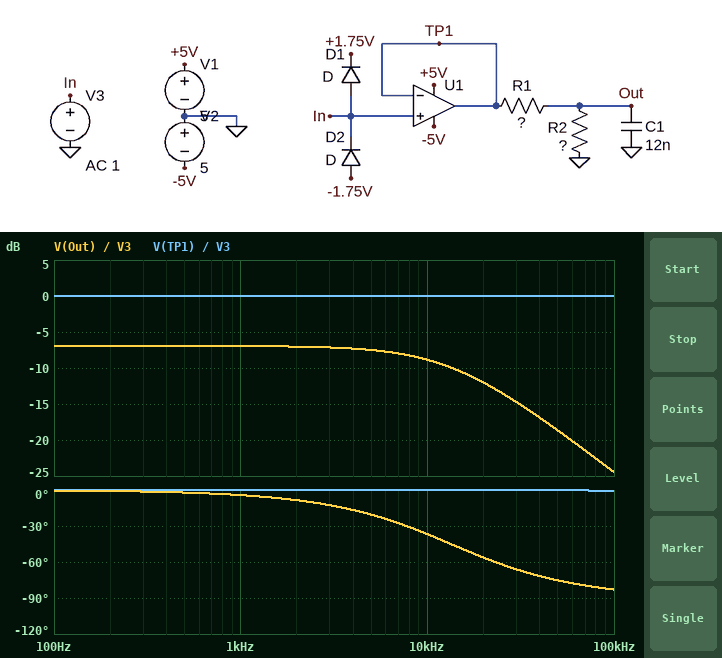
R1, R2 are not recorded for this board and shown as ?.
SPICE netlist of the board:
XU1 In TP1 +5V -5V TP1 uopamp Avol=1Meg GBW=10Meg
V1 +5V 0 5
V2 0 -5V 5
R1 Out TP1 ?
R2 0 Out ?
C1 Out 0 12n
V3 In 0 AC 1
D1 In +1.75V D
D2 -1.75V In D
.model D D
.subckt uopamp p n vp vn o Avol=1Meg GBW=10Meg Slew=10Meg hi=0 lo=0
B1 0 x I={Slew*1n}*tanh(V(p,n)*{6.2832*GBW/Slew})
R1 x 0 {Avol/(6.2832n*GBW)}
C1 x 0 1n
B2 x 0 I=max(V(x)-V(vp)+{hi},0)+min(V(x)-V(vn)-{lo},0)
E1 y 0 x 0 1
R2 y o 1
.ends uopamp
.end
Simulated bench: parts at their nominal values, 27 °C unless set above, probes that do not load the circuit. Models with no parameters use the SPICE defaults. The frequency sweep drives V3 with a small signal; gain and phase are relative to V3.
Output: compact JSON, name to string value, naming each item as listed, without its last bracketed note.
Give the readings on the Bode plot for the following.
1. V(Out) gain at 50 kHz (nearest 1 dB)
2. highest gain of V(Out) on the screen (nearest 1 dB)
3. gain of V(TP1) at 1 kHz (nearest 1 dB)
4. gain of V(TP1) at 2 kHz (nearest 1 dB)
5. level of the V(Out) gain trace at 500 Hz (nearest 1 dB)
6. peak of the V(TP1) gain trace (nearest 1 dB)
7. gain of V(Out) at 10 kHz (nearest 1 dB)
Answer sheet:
{"V(Out) gain at 50 kHz": "-19 dB", "highest gain of V(Out) on the screen": "-7 dB", "gain of V(TP1) at 1 kHz": "0 dB", "gain of V(TP1) at 2 kHz": "0 dB", "level of the V(Out) gain trace at 500 Hz": "-7 dB", "peak of the V(TP1) gain trace": "0 dB", "gain of V(Out) at 10 kHz": "-9 dB"}
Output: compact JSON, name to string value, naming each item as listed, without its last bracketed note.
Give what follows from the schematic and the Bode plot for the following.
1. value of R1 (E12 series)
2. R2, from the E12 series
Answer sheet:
{"value of R1": "2.2 kΩ", "R2, from the E12 series": "1.8 kΩ"}
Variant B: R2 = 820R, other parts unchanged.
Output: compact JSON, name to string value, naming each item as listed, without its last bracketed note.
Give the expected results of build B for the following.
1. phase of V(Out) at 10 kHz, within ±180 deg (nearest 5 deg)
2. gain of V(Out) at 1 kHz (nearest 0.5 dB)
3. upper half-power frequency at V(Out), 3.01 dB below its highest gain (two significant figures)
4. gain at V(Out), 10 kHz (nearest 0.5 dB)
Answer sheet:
{"phase of V(Out) at 10 kHz, within ±180 deg": "-25 deg", "gain of V(Out) at 1 kHz": "-11.5 dB", "upper half-power frequency at V(Out), 3.01 dB below its highest gain": "22 kHz", "gain at V(Out), 10 kHz": "-12.0 dB"}
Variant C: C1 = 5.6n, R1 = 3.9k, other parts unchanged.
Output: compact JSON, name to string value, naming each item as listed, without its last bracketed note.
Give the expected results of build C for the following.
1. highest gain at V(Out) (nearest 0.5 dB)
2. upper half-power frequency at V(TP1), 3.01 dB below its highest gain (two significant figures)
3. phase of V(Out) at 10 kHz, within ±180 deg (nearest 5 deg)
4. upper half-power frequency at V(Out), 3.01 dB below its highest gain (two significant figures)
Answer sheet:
{"highest gain at V(Out)": "-10.0 dB", "upper half-power frequency at V(TP1), 3.01 dB below its highest gain": "10 MHz", "phase of V(Out) at 10 kHz, within ±180 deg": "-25 deg", "upper half-power frequency at V(Out), 3.01 dB below its highest gain": "23 kHz"}
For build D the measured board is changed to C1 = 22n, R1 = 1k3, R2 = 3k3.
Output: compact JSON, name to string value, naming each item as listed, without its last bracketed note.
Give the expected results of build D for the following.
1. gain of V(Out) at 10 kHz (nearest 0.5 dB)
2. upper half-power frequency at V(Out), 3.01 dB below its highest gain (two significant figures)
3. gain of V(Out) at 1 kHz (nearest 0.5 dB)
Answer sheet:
{"gain of V(Out) at 10 kHz": "-7.0 dB", "upper half-power frequency at V(Out), 3.01 dB below its highest gain": "7.8 kHz", "gain of V(Out) at 1 kHz": "-3.0 dB"}
